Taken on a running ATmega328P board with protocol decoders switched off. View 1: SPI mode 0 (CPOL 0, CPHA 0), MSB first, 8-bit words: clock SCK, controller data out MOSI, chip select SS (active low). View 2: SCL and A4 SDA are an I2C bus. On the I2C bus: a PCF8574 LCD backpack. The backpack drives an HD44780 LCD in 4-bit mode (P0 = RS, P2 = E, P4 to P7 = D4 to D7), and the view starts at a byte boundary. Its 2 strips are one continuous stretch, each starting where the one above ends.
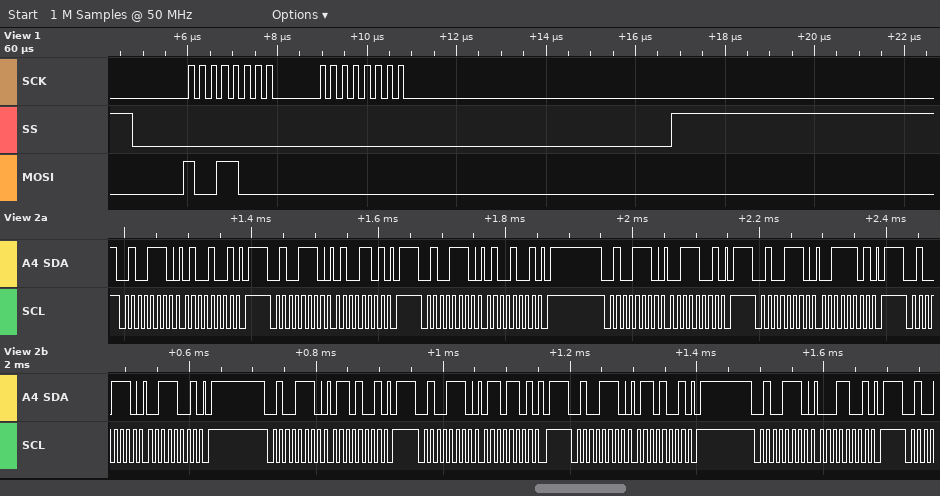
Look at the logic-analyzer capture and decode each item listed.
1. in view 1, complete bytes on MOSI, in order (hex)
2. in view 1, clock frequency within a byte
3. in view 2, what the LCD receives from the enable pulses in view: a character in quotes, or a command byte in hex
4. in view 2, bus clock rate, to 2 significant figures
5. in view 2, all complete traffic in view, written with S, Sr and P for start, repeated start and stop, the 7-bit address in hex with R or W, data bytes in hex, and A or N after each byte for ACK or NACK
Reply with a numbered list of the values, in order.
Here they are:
1. 0x98 0x00
2. 4 MHz
3. 'C'
4. 100 kHz
5. S 27W A 49 A P S 27W A 4D A P S 27W A 49 A P S 27W A 39 A P S 27W A 3D A P S 27W A 39 A P S 27W A 69 A P S 27W A 6D A P S 27W A 69 A P S 27W A 19 A P
